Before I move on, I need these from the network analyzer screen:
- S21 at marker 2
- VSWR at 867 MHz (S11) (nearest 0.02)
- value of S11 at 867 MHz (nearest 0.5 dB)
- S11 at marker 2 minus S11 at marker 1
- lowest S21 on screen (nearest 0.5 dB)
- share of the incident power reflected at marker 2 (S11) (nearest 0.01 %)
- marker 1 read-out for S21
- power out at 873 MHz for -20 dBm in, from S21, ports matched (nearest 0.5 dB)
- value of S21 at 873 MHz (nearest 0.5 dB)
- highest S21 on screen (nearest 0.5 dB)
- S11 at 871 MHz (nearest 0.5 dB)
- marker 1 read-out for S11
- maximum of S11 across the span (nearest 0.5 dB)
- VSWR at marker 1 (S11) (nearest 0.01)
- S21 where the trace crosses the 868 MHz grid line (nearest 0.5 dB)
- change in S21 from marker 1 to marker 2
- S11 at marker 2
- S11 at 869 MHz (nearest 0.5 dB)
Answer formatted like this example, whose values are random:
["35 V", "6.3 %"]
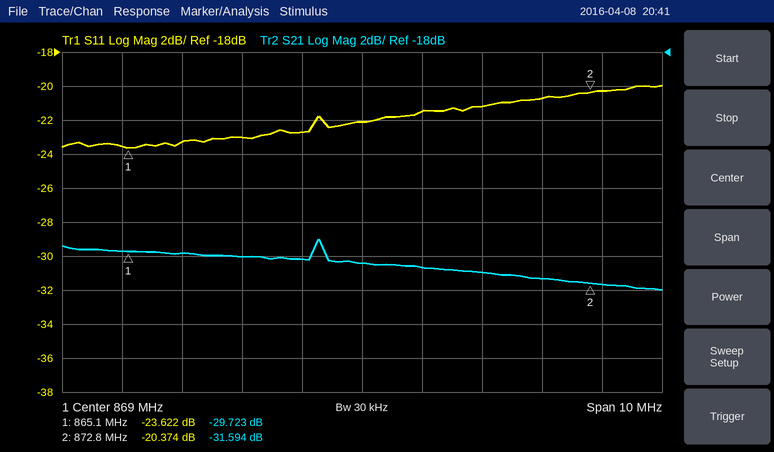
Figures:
["-31.594 dB", "1.16", "-23.0 dB", "3.248 dB", "-32.0 dB", "0.92 %", "-29.723 dB", "-51.5 dBm", "-31.5 dB", "-29.0 dB", "-21.0 dB", "-23.622 dB", "-20.0 dB", "1.14", "-30.0 dB", "-1.871 dB", "-20.374 dB", "-22.0 dB"]
